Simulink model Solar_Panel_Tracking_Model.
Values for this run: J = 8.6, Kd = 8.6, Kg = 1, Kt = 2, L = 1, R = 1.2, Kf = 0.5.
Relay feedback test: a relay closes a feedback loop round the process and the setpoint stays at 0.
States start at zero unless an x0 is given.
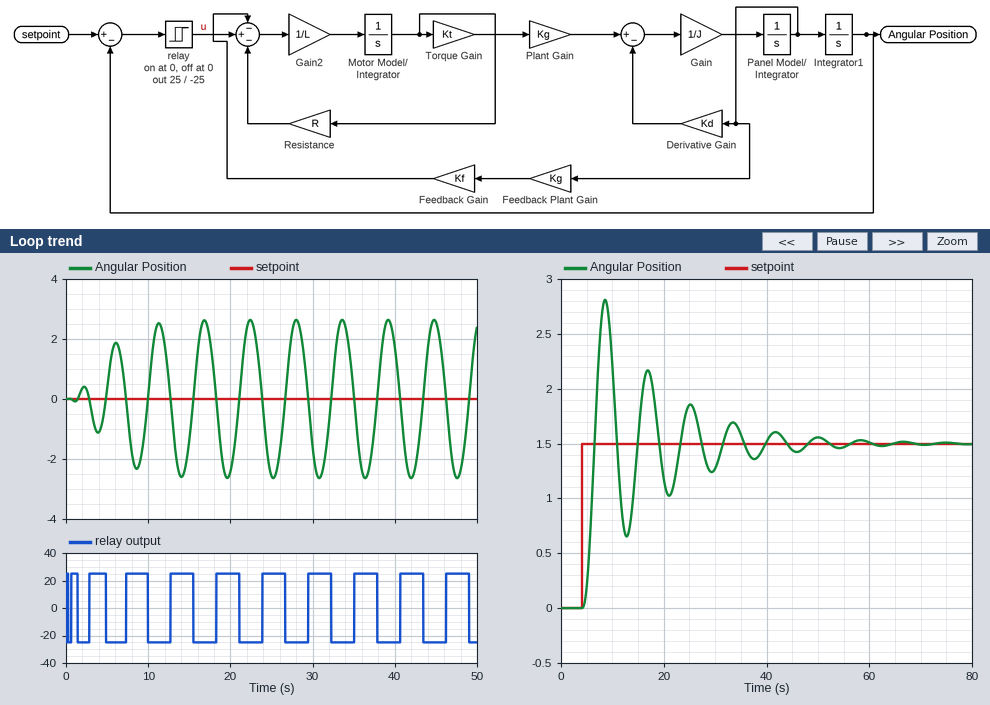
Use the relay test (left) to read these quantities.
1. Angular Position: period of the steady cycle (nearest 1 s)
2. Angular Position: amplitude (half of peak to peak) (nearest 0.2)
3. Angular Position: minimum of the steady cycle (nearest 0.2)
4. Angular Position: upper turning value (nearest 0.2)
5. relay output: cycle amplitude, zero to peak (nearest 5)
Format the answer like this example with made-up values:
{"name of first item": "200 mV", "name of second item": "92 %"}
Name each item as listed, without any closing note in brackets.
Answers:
{"Angular Position: period of the steady cycle": "6 s", "Angular Position: amplitude (half of peak to peak)": "2.6", "Angular Position: minimum of the steady cycle": "-2.6", "Angular Position: upper turning value": "2.6", "relay output: cycle amplitude, zero to peak": "25"}
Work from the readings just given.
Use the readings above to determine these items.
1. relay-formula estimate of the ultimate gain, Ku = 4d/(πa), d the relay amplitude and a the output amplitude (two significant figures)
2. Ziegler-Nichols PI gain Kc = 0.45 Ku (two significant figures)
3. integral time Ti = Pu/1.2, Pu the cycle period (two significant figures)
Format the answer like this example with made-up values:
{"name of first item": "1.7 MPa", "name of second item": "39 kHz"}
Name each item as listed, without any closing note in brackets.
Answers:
{"relay-formula estimate of the ultimate gain, Ku = 4d/(πa), d the relay amplitude and a the output amplitude": "12", "Ziegler-Nichols PI gain Kc = 0.45 Ku": "5.4", "integral time Ti = Pu/1.2, Pu the cycle period": "5.0 s"}
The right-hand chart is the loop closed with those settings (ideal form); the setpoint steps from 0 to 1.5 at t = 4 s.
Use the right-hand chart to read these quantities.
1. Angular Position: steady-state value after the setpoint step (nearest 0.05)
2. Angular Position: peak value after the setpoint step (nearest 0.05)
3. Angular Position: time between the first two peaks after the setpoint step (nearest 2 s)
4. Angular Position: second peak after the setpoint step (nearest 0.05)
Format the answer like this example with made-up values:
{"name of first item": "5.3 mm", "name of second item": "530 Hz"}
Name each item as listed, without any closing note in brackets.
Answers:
{"Angular Position: steady-state value after the setpoint step": "1.50", "Angular Position: peak value after the setpoint step": "2.80", "Angular Position: time between the first two peaks after the setpoint step": "8 s", "Angular Position: second peak after the setpoint step": "2.15"}
